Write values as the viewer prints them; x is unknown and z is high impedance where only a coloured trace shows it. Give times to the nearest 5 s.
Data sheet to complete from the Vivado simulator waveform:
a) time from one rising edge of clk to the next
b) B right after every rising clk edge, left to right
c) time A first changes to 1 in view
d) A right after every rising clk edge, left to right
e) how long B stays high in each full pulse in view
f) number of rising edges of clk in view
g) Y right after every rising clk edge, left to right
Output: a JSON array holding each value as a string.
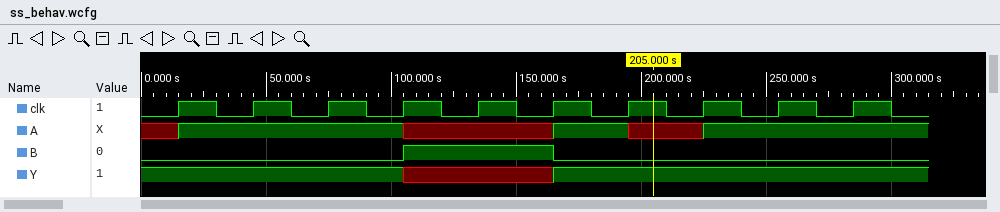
["30 s", "0 0 0 1 1 0 0 0 0 0", "15 s", "1 1 1 x x 1 x 1 1 1", "60 s", "10", "1 1 1 x x 1 1 1 1 1"]
